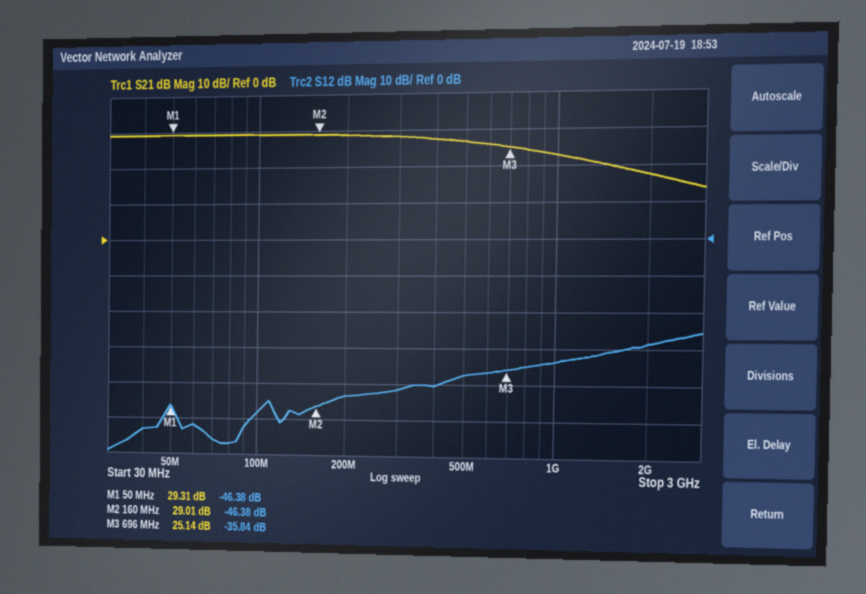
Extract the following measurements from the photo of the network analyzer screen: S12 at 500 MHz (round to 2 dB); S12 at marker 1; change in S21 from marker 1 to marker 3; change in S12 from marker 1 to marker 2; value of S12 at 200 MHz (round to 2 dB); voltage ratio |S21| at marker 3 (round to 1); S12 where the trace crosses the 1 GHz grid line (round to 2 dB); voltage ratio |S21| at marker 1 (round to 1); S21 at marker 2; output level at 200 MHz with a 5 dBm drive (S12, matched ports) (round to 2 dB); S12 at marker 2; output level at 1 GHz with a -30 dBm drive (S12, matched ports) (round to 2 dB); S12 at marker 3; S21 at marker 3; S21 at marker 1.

-38 dB
-46.38 dB
-4.17 dB
0.00 dB
-44 dB
18
-34 dB
29
29.01 dB
-38 dBm
-46.38 dB
-64 dBm
-35.84 dB
25.14 dB
29.31 dB
